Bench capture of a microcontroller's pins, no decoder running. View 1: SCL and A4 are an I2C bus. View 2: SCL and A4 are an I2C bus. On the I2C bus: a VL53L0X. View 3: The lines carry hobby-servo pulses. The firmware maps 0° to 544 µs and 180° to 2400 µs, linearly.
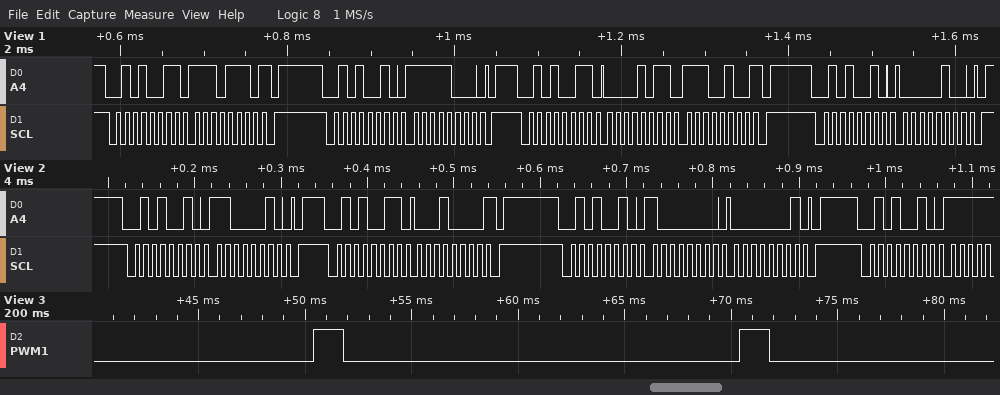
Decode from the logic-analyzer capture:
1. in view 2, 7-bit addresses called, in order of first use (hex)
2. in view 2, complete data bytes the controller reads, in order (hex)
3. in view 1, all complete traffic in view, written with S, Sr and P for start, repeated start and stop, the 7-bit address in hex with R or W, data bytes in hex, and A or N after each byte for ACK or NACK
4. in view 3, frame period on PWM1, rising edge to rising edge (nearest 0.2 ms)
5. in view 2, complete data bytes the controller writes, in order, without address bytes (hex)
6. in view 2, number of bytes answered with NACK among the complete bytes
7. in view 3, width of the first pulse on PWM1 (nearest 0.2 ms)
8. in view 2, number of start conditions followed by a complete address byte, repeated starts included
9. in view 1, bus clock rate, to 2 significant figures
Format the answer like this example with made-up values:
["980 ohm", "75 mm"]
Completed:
["0x29", "10", "S 29R A EE N P S 29W A F8 A P S 29R A 0B A E4 N P S 29W A 04 A P", "20.0 ms", "C2 80 01", "1", "1.4 ms", "4", "100 kHz"]
